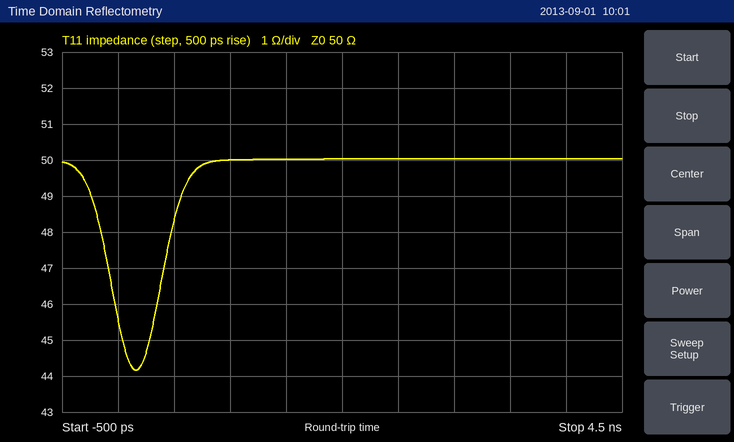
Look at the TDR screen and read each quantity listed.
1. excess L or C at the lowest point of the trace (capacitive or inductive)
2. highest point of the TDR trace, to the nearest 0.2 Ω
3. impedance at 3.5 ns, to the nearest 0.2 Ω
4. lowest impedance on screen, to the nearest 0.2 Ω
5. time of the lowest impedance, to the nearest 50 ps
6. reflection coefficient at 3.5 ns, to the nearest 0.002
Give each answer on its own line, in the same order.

capacitive
50.0 Ω
50.0 Ω
44.2 Ω
150 ps
0.000
